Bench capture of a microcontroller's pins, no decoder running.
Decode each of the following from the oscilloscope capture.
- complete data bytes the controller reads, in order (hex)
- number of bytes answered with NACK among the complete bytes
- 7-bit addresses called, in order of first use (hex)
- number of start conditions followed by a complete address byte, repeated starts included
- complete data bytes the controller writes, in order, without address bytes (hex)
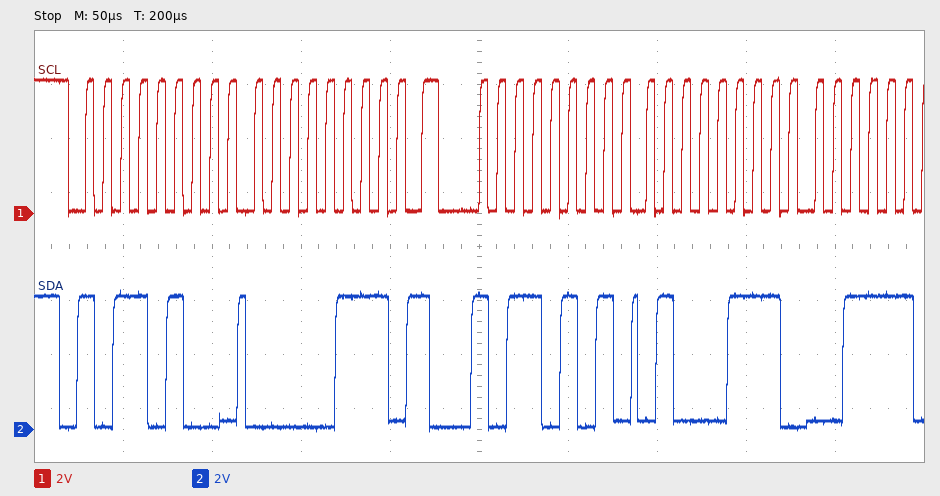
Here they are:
47
0
0x5A
2
07
